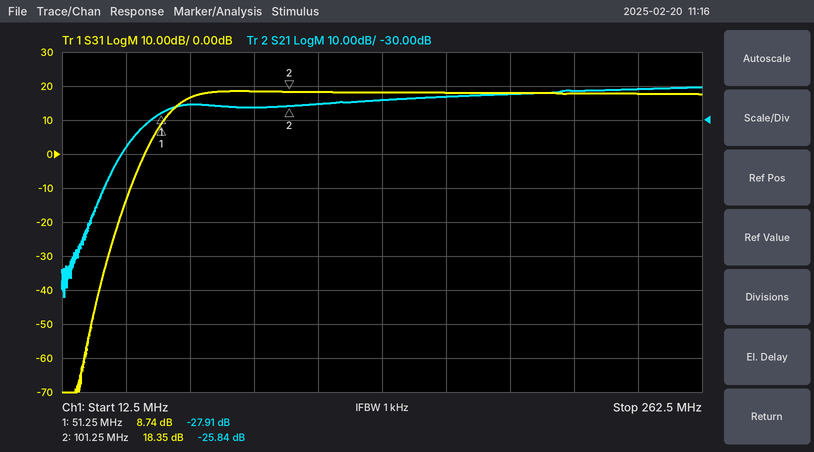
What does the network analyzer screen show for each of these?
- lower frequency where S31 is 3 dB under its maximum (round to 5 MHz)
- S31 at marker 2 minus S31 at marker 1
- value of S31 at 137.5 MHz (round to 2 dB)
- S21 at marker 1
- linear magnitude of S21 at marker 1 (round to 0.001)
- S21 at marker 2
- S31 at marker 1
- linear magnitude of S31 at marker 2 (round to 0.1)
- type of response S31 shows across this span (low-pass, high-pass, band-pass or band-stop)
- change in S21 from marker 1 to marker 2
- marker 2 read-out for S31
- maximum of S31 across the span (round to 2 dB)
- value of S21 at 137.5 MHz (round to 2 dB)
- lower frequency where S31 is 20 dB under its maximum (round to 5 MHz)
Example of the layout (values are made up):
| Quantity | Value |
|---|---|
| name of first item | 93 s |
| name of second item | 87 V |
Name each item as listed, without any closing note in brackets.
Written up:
| Quantity | Value |
|---|---|
| lower frequency where S31 is 3 dB under its maximum | 60 MHz |
| S31 at marker 2 minus S31 at marker 1 | 9.61 dB |
| value of S31 at 137.5 MHz | 18 dB |
| S21 at marker 1 | -27.91 dB |
| linear magnitude of S21 at marker 1 | 0.040 |
| S21 at marker 2 | -25.84 dB |
| S31 at marker 1 | 8.74 dB |
| linear magnitude of S31 at marker 2 | 8.3 |
| type of response S31 shows across this span | high-pass |
| change in S21 from marker 1 to marker 2 | 2.07 dB |
| marker 2 read-out for S31 | 18.35 dB |
| maximum of S31 across the span | 18 dB |
| value of S21 at 137.5 MHz | -24 dB |
| lower frequency where S31 is 20 dB under its maximum | 45 MHz |
